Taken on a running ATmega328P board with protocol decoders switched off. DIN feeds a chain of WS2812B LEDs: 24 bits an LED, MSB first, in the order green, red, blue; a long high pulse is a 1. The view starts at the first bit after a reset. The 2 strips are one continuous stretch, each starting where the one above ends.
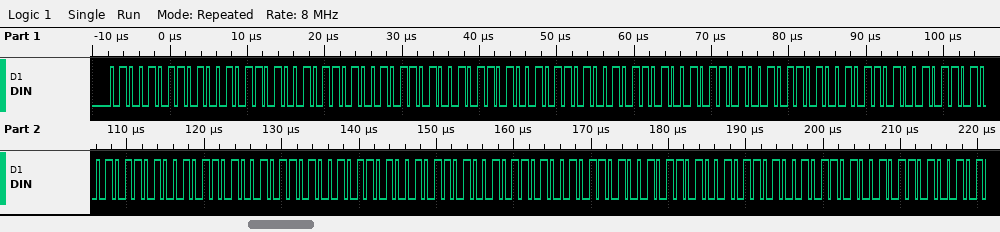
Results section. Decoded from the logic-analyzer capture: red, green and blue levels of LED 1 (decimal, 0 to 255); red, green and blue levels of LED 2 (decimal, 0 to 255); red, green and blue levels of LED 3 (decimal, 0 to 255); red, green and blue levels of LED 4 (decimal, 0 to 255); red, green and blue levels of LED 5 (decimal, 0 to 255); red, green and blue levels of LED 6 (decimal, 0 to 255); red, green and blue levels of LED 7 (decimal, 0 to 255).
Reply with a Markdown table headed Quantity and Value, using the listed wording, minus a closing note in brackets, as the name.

| Quantity | Value |
|---|---|
| red, green and blue levels of LED 1 | 75, 75, 75 |
| red, green and blue levels of LED 2 | 75, 75, 75 |
| red, green and blue levels of LED 3 | 75, 75, 75 |
| red, green and blue levels of LED 4 | 75, 75, 75 |
| red, green and blue levels of LED 5 | 75, 75, 75 |
| red, green and blue levels of LED 6 | 75, 75, 75 |
| red, green and blue levels of LED 7 | 75, 75, 75 |
